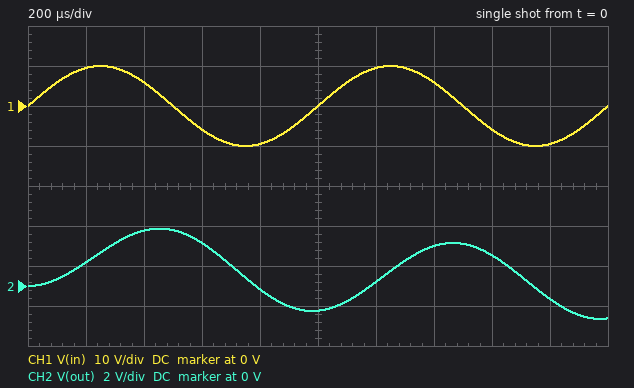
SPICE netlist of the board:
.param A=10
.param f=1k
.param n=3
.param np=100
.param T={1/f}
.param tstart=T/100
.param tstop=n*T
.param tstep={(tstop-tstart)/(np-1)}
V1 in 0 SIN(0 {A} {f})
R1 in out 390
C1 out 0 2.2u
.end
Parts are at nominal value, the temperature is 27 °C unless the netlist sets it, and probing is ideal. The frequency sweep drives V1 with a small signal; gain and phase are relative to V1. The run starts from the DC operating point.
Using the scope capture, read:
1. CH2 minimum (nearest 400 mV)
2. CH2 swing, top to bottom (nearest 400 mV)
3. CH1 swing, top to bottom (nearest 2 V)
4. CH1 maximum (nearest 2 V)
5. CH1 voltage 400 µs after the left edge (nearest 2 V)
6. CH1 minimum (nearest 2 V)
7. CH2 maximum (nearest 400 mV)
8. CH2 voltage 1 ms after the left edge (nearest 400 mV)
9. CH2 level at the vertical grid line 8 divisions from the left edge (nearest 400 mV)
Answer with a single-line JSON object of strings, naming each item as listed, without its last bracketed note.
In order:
{"CH2 minimum": "-1.6 V", "CH2 swing, top to bottom": "4.4 V", "CH1 swing, top to bottom": "20 V", "CH1 maximum": "10 V", "CH1 voltage 400 µs after the left edge": "6 V", "CH1 minimum": "-10 V", "CH2 maximum": "2.8 V", "CH2 voltage 1 ms after the left edge": "-1.2 V", "CH2 level at the vertical grid line 8 divisions from the left edge": "1.6 V"}
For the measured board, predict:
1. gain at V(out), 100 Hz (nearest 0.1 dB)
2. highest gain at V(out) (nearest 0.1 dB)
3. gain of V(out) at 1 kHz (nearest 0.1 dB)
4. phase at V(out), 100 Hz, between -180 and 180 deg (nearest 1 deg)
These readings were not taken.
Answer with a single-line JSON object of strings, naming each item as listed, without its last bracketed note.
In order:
{"gain at V(out), 100 Hz": "-1.1 dB", "highest gain at V(out)": "0 dB", "gain of V(out) at 1 kHz": "-14.8 dB", "phase at V(out), 100 Hz, between -180 and 180 deg": "-28 deg"}
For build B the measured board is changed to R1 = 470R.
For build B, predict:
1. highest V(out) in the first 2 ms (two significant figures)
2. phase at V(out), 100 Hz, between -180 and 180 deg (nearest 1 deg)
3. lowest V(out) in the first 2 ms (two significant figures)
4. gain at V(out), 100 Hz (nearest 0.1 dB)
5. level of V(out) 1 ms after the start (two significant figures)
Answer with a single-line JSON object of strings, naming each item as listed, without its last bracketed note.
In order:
{"highest V(out) in the first 2 ms": "2.5 V", "phase at V(out), 100 Hz, between -180 and 180 deg": "-33 deg", "lowest V(out) in the first 2 ms": "-1.3 V", "gain at V(out), 100 Hz": "-1.5 dB", "level of V(out) 1 ms after the start": "-930 mV"}
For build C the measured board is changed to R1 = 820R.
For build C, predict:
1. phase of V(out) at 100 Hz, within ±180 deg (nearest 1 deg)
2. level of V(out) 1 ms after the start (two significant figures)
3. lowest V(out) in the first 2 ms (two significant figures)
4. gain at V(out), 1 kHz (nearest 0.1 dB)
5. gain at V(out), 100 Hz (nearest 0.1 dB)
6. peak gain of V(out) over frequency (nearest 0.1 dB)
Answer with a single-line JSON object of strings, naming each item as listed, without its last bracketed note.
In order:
{"phase of V(out) at 100 Hz, within ±180 deg": "-49 deg", "level of V(out) 1 ms after the start": "-370 mV", "lowest V(out) in the first 2 ms": "-590 mV", "gain at V(out), 1 kHz": "-21.1 dB", "gain at V(out), 100 Hz": "-3.6 dB", "peak gain of V(out) over frequency": "0 dB"}
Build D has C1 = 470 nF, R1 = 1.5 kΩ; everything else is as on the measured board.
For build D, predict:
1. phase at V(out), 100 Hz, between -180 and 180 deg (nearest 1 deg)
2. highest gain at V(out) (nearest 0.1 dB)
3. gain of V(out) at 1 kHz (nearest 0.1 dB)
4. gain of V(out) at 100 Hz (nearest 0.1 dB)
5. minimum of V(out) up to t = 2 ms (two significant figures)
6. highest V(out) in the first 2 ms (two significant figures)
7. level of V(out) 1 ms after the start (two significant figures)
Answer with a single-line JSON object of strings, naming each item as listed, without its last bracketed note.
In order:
{"phase at V(out), 100 Hz, between -180 and 180 deg": "-24 deg", "highest gain at V(out)": "0 dB", "gain of V(out) at 1 kHz": "-13.1 dB", "gain of V(out) at 100 Hz": "-0.8 dB", "minimum of V(out) up to t = 2 ms": "-2.1 V", "highest V(out) in the first 2 ms": "3.3 V", "level of V(out) 1 ms after the start": "-1.6 V"}
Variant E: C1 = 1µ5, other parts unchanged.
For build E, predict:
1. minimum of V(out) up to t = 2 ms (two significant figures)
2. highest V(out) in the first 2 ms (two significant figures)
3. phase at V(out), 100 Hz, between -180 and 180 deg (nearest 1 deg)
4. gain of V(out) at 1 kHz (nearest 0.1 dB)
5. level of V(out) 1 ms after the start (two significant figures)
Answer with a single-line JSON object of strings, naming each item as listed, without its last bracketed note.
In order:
{"minimum of V(out) up to t = 2 ms": "-2.5 V", "highest V(out) in the first 2 ms": "3.8 V", "phase at V(out), 100 Hz, between -180 and 180 deg": "-20 deg", "gain of V(out) at 1 kHz": "-11.6 dB", "level of V(out) 1 ms after the start": "-2.1 V"}
